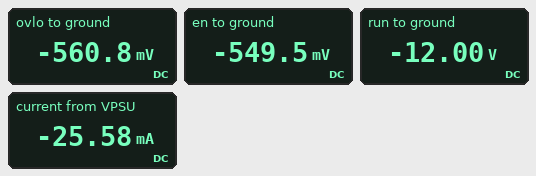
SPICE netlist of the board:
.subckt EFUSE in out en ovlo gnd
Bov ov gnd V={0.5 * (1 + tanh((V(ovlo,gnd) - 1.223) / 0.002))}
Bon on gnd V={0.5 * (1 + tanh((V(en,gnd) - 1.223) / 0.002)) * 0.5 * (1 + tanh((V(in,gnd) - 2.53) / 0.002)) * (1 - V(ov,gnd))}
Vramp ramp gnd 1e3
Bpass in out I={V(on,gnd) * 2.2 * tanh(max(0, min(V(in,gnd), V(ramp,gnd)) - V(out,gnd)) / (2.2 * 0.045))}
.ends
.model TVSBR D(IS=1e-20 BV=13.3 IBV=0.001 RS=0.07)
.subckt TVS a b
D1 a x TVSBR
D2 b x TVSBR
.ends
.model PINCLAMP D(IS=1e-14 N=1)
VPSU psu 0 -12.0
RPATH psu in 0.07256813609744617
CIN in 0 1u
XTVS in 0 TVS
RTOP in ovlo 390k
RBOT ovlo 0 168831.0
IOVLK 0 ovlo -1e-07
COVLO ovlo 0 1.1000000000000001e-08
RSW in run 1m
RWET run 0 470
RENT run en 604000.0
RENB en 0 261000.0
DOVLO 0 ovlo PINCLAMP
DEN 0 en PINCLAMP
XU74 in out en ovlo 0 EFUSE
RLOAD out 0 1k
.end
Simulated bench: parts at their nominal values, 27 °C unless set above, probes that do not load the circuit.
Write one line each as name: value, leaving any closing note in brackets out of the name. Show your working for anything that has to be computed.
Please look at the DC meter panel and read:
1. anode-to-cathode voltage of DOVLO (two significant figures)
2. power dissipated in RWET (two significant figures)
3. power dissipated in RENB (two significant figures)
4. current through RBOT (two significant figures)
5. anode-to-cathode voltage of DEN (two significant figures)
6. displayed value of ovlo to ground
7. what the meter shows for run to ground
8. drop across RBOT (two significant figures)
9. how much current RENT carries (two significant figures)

anode-to-cathode voltage of DOVLO: 0 V - (-560.8 mV) = 560 mV
power dissipated in RWET: (0 V - (-12 V))^2 / 470 Ω = 310 mW
power dissipated in RENB: (0 V - (-549.5 mV))^2 / 261 kΩ = 1.2 µW
current through RBOT: (0 V - (-560.8 mV)) / 168.8 kΩ = 3.3 µA
anode-to-cathode voltage of DEN: 0 V - (-549.5 mV) = 550 mV
displayed value of ovlo to ground: -560.8 mV
what the meter shows for run to ground: -12.00 V
drop across RBOT: 0 V - (-560.8 mV) = 560 mV
how much current RENT carries: (-549.5 mV - (-12 V)) / 604 kΩ = 19 µA
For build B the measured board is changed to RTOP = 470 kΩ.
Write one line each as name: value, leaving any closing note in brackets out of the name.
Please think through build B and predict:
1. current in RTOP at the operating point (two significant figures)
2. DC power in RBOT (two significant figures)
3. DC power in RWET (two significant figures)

current in RTOP at the operating point: 24 µA
DC power in RBOT: 1.8 µW
DC power in RWET: 310 mW
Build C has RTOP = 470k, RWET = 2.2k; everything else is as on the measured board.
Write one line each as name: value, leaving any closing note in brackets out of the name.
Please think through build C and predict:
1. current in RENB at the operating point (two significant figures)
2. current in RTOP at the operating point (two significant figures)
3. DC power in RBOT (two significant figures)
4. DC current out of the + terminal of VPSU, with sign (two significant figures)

current in RENB at the operating point: 2.1 µA
current in RTOP at the operating point: 24 µA
DC power in RBOT: 1.8 µW
DC current out of the + terminal of VPSU, with sign: -5.5 mA
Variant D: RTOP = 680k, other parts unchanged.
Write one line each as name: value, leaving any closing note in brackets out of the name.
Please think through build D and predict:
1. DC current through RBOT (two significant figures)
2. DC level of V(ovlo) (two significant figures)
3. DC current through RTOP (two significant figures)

DC current through RBOT: 3.2 µA
DC level of V(ovlo): -540 mV
DC current through RTOP: 17 µA
